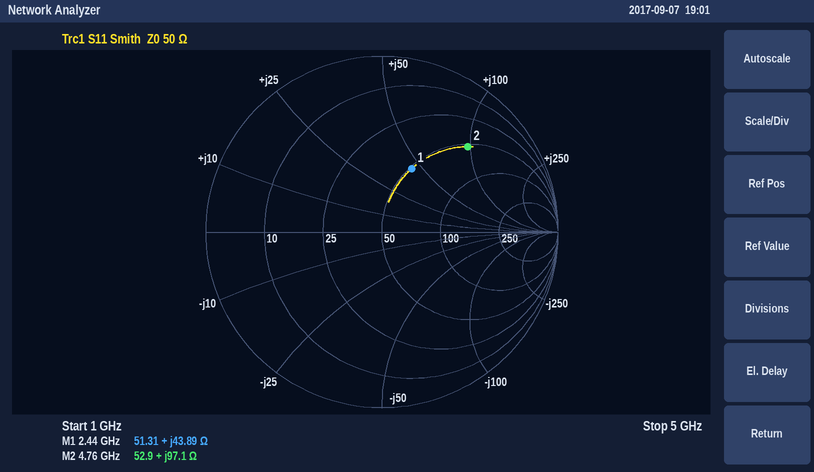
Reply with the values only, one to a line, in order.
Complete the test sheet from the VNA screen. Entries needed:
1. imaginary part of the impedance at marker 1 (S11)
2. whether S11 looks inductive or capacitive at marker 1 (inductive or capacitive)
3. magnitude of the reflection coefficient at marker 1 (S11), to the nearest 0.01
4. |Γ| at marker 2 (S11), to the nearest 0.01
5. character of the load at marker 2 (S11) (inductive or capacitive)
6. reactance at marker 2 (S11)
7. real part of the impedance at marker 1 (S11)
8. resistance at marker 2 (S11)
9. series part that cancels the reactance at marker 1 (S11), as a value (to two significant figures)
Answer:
+43.89 Ω
inductive
0.40
0.69
inductive
+97.1 Ω
51.31 Ω
52.9 Ω
1.5 pF
